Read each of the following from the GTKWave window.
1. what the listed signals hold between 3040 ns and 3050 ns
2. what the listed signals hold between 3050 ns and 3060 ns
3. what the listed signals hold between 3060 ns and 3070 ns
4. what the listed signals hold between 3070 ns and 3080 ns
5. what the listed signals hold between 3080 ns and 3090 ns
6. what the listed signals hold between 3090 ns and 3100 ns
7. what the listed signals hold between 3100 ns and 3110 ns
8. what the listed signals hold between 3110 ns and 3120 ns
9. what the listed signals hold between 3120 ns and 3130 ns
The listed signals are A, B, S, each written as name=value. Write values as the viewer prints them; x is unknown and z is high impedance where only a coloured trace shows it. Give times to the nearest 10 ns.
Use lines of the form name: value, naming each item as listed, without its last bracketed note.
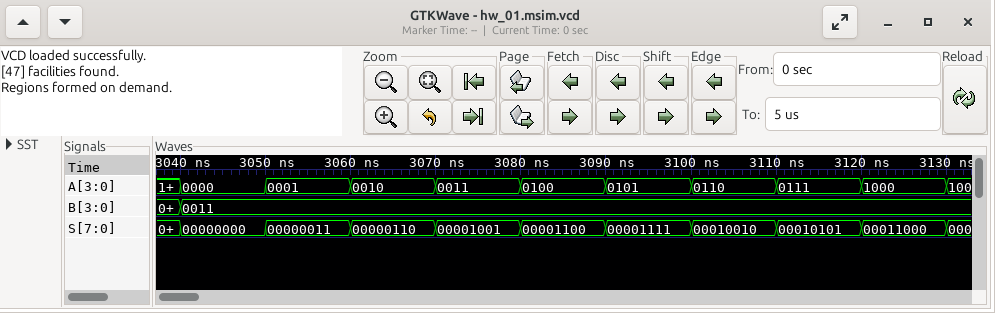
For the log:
what the listed signals hold between 3040 ns and 3050 ns: A=0000, B=0011, S=00000000
what the listed signals hold between 3050 ns and 3060 ns: A=0001, B=0011, S=00000011
what the listed signals hold between 3060 ns and 3070 ns: A=0010, B=0011, S=00000110
what the listed signals hold between 3070 ns and 3080 ns: A=0011, B=0011, S=00001001
what the listed signals hold between 3080 ns and 3090 ns: A=0100, B=0011, S=00001100
what the listed signals hold between 3090 ns and 3100 ns: A=0101, B=0011, S=00001111
what the listed signals hold between 3100 ns and 3110 ns: A=0110, B=0011, S=00010010
what the listed signals hold between 3110 ns and 3120 ns: A=0111, B=0011, S=00010101
what the listed signals hold between 3120 ns and 3130 ns: A=1000, B=0011, S=00011000
